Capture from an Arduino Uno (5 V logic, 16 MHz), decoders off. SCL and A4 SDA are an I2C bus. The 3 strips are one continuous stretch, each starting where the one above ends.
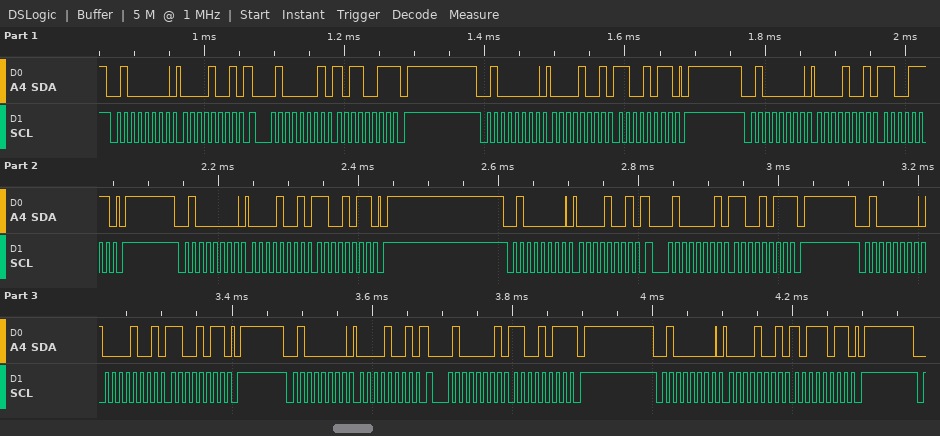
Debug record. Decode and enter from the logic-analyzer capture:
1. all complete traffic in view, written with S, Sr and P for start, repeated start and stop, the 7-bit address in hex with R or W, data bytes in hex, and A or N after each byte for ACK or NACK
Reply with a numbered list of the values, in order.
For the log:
1. S 20W A 09 A Sr 20R A B3 N P S 20W A 09 A CB A P S 20W A 09 A CF A P S 20W A 09 A CB A P S 20W A 09 A Sr 20R A CB N P S 20W A 09 A CB A P S 20W A 09 A Sr 20R A CB N P S 20W A 09 A BB A P
